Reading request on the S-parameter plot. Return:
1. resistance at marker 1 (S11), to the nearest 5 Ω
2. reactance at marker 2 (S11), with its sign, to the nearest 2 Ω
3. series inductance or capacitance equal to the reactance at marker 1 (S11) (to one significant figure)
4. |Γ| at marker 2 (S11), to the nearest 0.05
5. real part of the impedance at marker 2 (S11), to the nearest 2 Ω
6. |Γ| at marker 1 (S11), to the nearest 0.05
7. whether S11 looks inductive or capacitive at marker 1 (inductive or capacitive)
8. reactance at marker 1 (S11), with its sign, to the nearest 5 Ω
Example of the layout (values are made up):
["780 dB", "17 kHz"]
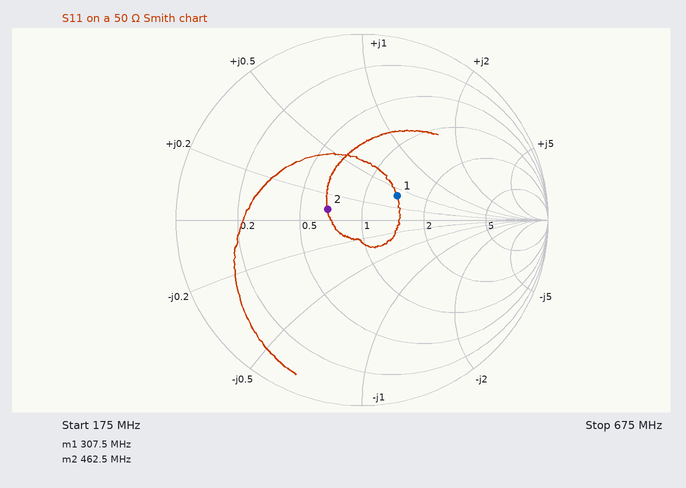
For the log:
["70 Ω", "+4 Ω", "10 nH", "0.20", "34 Ω", "0.25", "inductive", "+20 Ω"]
